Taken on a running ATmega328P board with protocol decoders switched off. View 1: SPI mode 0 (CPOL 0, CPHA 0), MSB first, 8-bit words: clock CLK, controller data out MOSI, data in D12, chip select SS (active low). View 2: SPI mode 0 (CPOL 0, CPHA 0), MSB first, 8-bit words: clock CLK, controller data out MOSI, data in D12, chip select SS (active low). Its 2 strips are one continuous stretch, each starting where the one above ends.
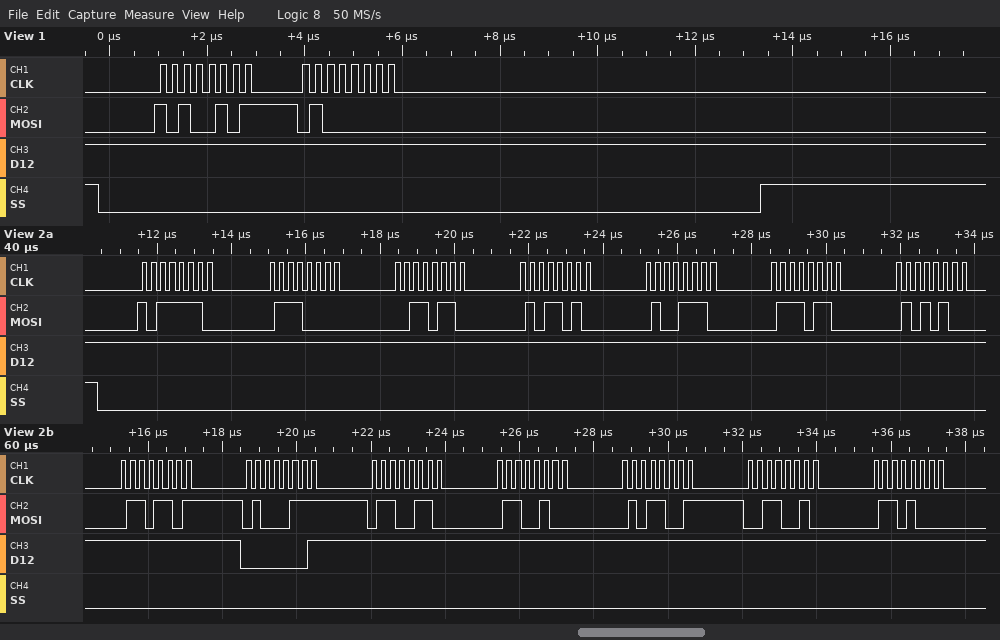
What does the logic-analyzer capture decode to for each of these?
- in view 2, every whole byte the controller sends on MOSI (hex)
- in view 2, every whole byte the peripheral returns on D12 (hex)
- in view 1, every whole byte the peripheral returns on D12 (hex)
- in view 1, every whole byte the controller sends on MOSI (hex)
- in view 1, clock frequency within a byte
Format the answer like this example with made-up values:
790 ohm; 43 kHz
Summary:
BE 70 36 5A 4E 76 54 6D 47 66 64 59 32 68; FF FF FF FF FF FF FF FF 01 FF FF FF FF FF; FF FF; A5 40; 4 MHz
